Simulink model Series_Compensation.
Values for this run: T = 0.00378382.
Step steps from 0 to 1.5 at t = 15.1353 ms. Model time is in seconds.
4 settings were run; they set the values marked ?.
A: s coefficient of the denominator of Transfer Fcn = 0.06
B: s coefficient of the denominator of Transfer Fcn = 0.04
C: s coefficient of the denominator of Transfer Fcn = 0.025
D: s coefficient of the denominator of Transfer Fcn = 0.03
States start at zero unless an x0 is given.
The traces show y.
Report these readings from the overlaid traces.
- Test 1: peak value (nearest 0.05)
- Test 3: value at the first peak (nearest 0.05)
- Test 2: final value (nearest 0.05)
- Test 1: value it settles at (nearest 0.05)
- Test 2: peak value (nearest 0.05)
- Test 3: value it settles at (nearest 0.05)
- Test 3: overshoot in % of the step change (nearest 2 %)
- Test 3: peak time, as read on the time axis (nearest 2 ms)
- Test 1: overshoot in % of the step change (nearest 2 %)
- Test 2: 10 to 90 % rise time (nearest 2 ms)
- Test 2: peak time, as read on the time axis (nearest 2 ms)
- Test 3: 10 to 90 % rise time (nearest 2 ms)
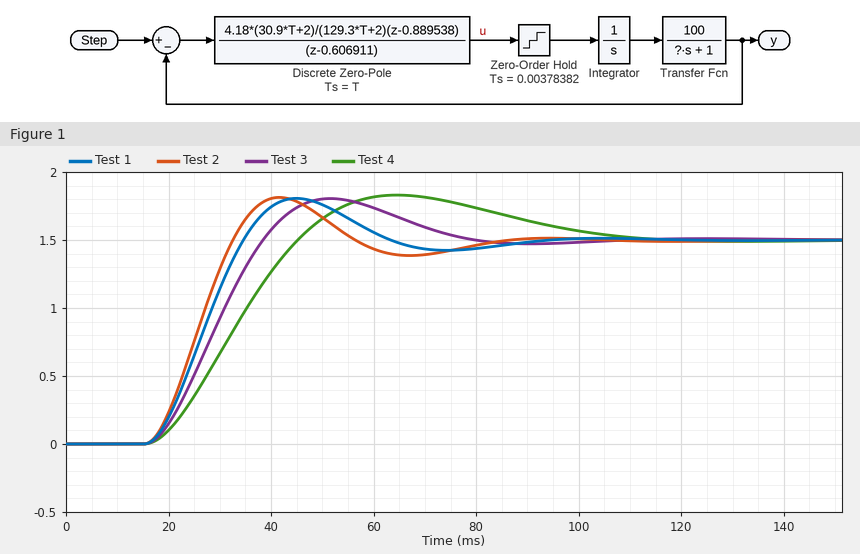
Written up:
1.80
1.80
1.50
1.50
1.80
1.50
20 %
52 ms
20 %
12 ms
42 ms
16 ms
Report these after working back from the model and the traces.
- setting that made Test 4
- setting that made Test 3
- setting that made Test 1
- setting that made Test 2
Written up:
A
B
D
C
